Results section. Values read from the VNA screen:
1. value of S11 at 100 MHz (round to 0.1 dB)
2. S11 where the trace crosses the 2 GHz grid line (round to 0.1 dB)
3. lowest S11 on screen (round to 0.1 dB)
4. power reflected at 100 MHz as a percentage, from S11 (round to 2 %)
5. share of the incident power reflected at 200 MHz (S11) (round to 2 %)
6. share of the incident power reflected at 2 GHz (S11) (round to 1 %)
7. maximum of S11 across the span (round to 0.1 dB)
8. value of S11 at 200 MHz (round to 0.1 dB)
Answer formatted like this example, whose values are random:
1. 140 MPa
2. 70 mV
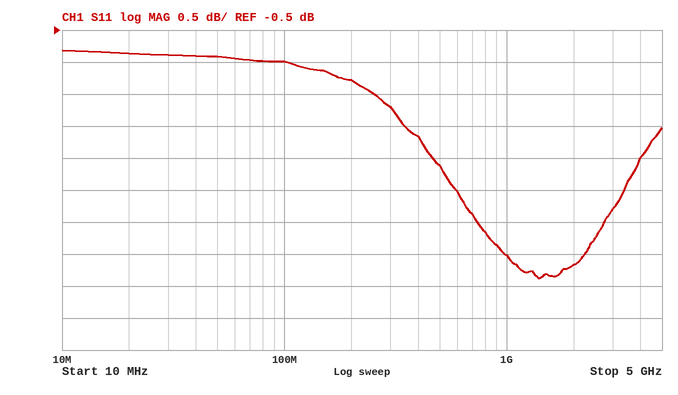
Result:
1. -1.0 dB
2. -4.2 dB
3. -4.4 dB
4. 80 %
5. 74 %
6. 38 %
7. -0.8 dB
8. -1.3 dB
